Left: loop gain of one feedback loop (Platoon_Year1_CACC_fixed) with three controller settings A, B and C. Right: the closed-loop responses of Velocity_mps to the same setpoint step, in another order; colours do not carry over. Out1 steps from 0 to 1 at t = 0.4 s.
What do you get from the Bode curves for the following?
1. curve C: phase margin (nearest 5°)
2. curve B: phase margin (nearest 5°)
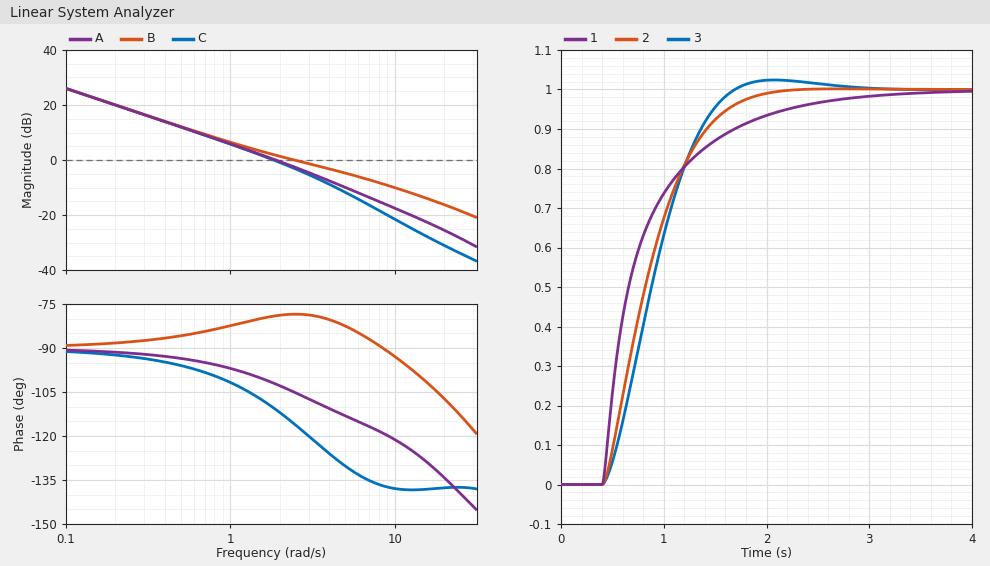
70°
100°
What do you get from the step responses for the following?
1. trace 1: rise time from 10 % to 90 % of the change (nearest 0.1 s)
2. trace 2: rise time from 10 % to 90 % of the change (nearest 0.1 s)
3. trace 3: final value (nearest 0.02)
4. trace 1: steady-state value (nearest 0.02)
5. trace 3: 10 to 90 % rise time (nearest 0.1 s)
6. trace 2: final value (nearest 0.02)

1.2 s
0.9 s
1.00
1.00
0.8 s
1.00
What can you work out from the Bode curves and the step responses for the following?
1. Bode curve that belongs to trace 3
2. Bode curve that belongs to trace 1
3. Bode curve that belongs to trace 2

C
B
A
